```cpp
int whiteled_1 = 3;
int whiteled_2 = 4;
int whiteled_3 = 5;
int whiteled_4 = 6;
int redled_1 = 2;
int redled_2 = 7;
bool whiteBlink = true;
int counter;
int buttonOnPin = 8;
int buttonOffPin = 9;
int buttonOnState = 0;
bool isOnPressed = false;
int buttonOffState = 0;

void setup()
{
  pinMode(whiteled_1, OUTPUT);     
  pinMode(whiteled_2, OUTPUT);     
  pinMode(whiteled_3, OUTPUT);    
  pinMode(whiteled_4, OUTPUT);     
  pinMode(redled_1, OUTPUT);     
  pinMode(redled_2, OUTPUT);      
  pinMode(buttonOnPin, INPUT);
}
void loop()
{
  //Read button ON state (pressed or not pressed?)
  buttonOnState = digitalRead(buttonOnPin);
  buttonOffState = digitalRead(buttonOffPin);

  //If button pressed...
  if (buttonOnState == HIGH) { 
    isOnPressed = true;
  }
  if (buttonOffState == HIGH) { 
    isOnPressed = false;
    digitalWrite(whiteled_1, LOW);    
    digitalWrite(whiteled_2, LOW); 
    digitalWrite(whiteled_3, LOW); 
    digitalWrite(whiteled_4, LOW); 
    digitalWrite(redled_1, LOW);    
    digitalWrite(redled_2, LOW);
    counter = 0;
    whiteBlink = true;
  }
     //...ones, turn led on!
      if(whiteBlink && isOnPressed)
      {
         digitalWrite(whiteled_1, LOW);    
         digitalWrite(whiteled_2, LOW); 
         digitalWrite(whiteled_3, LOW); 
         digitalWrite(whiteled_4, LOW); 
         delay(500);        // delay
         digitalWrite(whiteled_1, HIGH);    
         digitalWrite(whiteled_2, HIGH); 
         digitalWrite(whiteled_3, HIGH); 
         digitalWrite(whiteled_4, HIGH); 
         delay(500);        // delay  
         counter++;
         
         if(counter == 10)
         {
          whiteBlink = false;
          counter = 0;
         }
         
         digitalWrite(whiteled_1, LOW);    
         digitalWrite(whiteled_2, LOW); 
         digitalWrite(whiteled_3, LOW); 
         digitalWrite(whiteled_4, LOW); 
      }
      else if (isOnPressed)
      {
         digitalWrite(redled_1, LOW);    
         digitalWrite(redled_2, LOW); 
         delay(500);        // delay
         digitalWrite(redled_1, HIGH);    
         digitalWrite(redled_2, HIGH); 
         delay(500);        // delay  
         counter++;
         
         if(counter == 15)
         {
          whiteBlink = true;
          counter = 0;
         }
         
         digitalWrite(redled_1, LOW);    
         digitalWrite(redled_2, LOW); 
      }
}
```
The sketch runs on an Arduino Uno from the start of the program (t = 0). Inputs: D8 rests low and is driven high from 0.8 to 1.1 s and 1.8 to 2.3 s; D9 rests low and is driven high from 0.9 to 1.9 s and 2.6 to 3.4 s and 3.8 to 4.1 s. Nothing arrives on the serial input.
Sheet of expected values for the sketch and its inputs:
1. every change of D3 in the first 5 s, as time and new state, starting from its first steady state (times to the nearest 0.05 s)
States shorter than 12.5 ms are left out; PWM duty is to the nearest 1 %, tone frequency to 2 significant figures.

0 s low; 1.3 s high; 1.8 s low; 2.4 s high; 2.9 s low
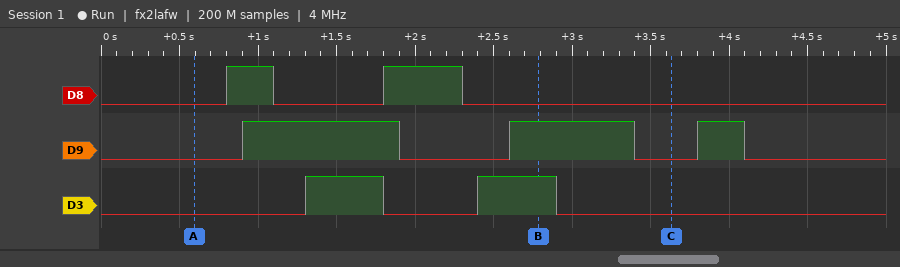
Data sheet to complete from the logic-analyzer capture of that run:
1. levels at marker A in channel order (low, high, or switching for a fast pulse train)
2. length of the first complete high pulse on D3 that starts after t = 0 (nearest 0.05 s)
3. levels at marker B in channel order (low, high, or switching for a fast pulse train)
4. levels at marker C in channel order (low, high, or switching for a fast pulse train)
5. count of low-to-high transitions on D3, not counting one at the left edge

D8 low, D9 low, D3 low
0.50 s
D8 low, D9 high, D3 high
D8 low, D9 low, D3 low
2
